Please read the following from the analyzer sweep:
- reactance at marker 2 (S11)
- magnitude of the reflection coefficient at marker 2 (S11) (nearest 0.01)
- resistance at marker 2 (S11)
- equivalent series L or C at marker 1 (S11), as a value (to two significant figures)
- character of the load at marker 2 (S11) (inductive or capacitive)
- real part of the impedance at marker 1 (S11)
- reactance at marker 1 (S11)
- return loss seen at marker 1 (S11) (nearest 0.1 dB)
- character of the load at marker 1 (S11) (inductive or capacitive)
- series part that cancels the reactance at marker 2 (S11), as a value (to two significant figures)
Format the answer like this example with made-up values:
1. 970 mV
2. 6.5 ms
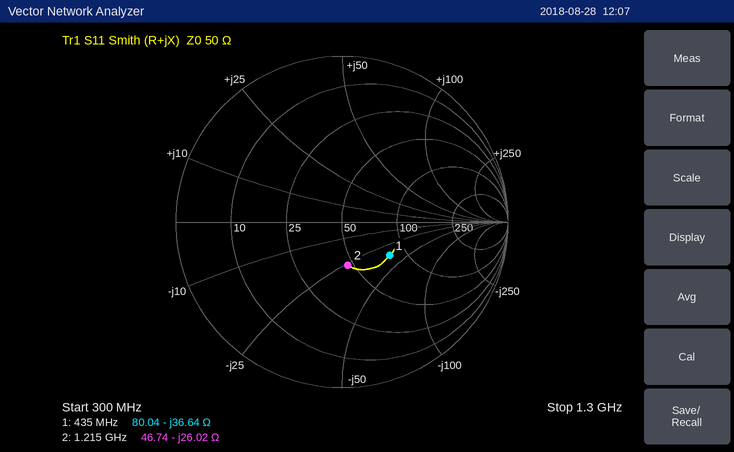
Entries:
1. -26.02 Ω
2. 0.26
3. 46.74 Ω
4. 10.0 pF
5. capacitive
6. 80.04 Ω
7. -36.64 Ω
8. 9.1 dB
9. capacitive
10. 3.4 nH
